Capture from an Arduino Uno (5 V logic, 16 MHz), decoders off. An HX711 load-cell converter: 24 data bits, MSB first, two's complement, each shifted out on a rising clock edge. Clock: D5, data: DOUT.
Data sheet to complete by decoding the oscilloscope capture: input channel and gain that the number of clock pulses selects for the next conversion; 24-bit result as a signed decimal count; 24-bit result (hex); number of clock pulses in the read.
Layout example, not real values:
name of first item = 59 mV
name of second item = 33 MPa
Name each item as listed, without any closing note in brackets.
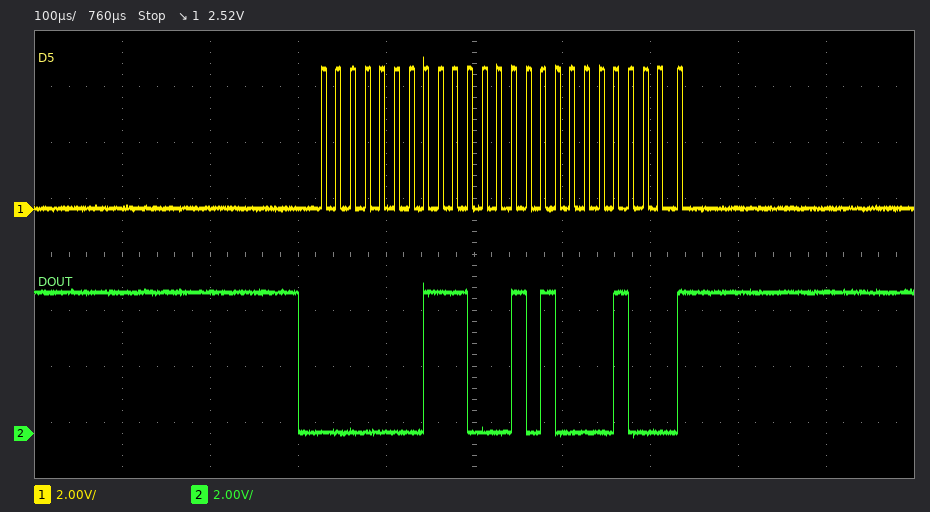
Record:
input channel and gain that the number of clock pulses selects for the next conversion = channel A, gain 128
24-bit result as a signed decimal count = 115976
24-bit result = 0x01C508
number of clock pulses in the read = 25
